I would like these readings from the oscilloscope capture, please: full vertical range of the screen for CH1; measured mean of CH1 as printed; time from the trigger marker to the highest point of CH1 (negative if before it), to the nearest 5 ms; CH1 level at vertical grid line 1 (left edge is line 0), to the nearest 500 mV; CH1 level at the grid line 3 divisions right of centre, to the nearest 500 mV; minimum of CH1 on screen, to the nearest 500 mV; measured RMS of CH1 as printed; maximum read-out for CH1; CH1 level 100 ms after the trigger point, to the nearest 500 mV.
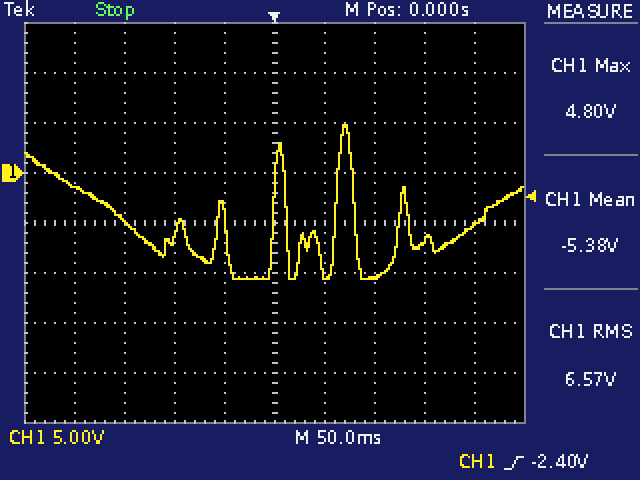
40 V
-5.38 V
+70 ms
-1.5 V
-6.5 V
-10.5 V
6.57 V
4.80 V
-10.5 V
